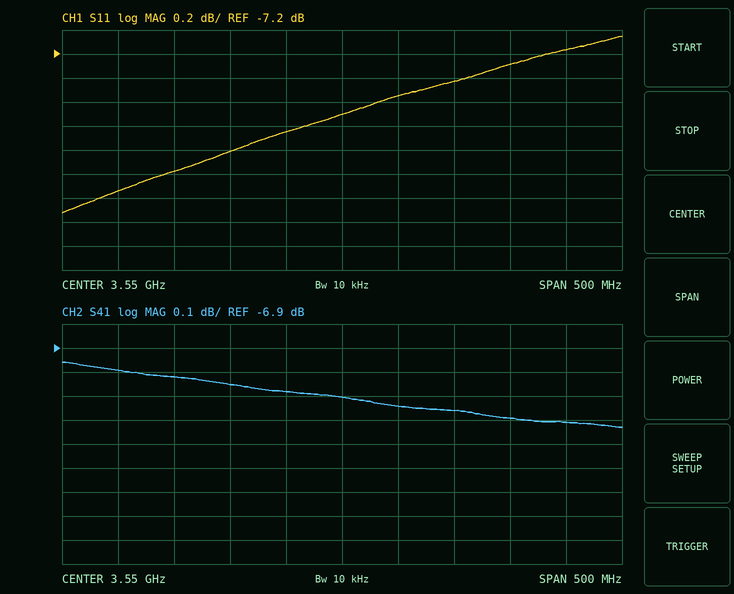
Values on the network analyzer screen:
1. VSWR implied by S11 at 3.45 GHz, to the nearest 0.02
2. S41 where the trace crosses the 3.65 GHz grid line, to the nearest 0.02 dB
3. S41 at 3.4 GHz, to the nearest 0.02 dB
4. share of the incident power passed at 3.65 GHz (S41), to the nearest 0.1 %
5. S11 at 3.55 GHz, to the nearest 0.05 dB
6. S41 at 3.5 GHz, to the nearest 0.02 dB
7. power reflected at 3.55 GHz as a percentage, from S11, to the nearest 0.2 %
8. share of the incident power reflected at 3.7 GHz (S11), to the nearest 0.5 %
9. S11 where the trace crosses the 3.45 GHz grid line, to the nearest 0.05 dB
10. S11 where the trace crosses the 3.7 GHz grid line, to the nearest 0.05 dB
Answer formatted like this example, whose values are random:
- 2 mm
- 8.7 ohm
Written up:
- 2.32
- -7.16 dB
- -7.02 dB
- 19.2 %
- -7.70 dB
- -7.08 dB
- 17.0 %
- 18.5 %
- -8.00 dB
- -7.30 dB
